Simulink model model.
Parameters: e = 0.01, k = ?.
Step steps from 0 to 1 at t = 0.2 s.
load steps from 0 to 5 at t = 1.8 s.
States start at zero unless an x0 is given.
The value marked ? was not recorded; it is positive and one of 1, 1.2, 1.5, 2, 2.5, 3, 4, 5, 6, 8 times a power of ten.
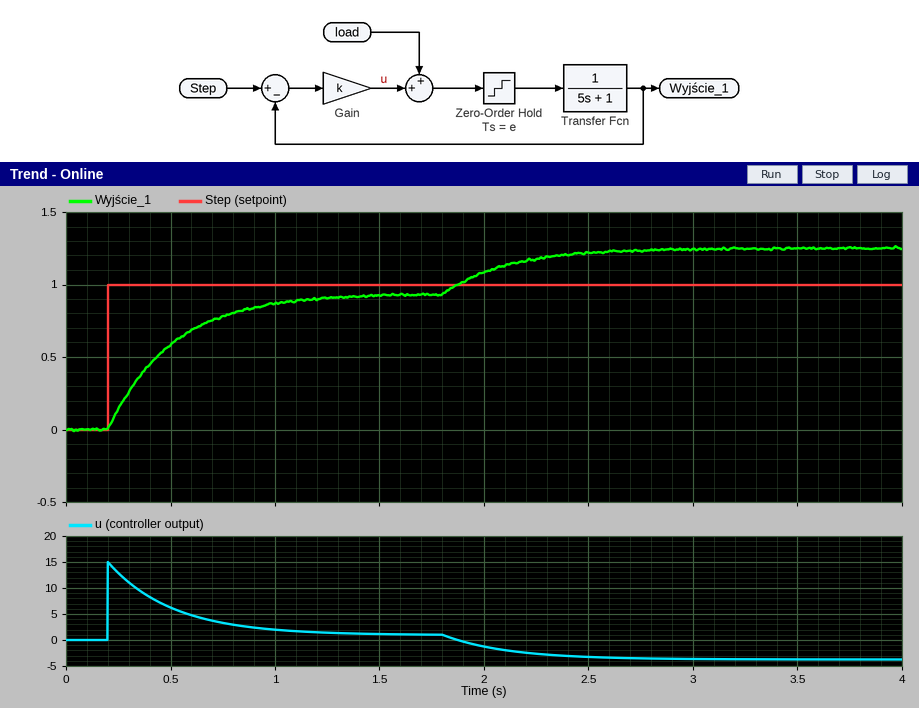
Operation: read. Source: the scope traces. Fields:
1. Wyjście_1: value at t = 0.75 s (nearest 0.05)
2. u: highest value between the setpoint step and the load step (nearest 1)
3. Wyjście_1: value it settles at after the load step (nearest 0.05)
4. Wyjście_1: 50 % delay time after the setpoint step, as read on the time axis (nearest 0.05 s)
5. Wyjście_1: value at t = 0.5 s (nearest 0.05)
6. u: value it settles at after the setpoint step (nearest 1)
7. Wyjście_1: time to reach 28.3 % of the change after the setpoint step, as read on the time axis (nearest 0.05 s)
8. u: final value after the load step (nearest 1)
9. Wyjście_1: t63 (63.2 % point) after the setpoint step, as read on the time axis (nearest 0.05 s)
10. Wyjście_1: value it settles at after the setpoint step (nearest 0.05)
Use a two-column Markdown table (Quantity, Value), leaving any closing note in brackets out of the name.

| Quantity | Value |
|---|---|
| Wyjście_1: value at t = 0.75 s | 0.80 |
| u: highest value between the setpoint step and the load step | 15 |
| Wyjście_1: value it settles at after the load step | 1.25 |
| Wyjście_1: 50 % delay time after the setpoint step, as read on the time axis | 0.40 s |
| Wyjście_1: value at t = 0.5 s | 0.60 |
| u: value it settles at after the setpoint step | 1 |
| Wyjście_1: time to reach 28.3 % of the change after the setpoint step, as read on the time axis | 0.30 s |
| u: final value after the load step | -4 |
| Wyjście_1: t63 (63.2 % point) after the setpoint step, as read on the time axis | 0.50 s |
| Wyjście_1: value it settles at after the setpoint step | 0.95 |
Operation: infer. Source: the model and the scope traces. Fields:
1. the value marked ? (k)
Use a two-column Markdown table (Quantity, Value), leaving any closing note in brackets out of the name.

| Quantity | Value |
|---|---|
| the value marked ? | 15 |
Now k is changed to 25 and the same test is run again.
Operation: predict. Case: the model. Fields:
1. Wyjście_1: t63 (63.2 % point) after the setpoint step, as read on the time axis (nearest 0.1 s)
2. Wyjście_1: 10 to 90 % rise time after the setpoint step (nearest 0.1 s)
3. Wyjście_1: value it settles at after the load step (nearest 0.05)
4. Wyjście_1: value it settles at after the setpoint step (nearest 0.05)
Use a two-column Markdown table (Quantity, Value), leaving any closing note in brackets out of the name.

| Quantity | Value |
|---|---|
| Wyjście_1: t63 (63.2 % point) after the setpoint step, as read on the time axis | 0.4 s |
| Wyjście_1: 10 to 90 % rise time after the setpoint step | 0.4 s |
| Wyjście_1: value it settles at after the load step | 1.15 |
| Wyjście_1: value it settles at after the setpoint step | 0.95 |
